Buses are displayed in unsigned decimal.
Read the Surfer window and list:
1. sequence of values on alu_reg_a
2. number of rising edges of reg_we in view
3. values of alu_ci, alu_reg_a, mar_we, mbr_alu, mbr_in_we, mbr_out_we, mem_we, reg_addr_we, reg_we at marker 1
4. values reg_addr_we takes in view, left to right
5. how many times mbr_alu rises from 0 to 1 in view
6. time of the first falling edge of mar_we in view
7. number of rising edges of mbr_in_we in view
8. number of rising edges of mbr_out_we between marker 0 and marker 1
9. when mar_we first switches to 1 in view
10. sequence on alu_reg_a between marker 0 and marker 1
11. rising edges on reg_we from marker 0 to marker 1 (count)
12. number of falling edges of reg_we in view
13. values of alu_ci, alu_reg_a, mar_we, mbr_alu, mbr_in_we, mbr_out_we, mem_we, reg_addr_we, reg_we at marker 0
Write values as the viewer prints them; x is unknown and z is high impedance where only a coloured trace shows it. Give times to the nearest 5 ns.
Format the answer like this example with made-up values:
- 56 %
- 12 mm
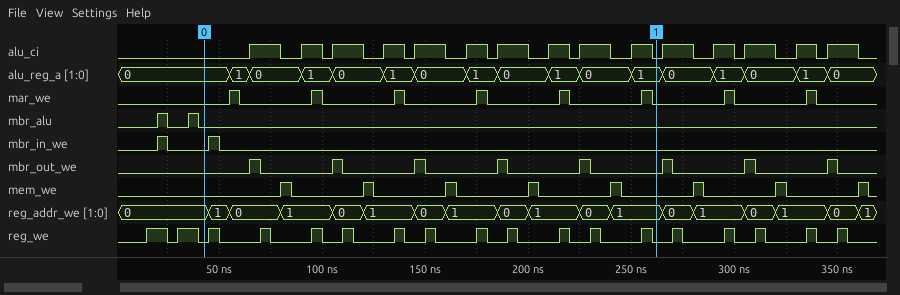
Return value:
- 0, 1, 0, 1, 0, 1, 0, 1, 0, 1, 0, 1, 0, 1, 0, 1, 0
- 18
- alu_ci=0, alu_reg_a=1, mar_we=0, mbr_alu=0, mbr_in_we=0, mbr_out_we=0, mem_we=0, reg_addr_we=1, reg_we=0
- 0, 1, 0, 1, 0, 1, 0, 1, 0, 1, 0, 1, 0, 1, 0, 1, 0, 1
- 2
- 60 ns
- 2
- 5
- 55 ns
- 0, 1, 0, 1, 0, 1, 0, 1, 0, 1, 0, 1
- 11
- 18
- alu_ci=0, alu_reg_a=0, mar_we=0, mbr_alu=0, mbr_in_we=0, mbr_out_we=0, mem_we=0, reg_addr_we=0, reg_we=0
